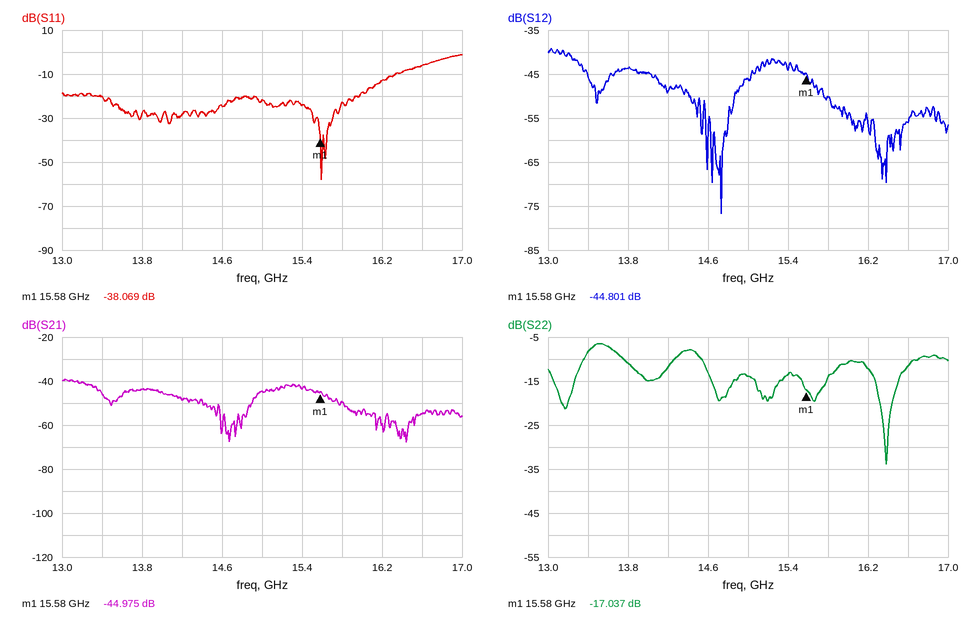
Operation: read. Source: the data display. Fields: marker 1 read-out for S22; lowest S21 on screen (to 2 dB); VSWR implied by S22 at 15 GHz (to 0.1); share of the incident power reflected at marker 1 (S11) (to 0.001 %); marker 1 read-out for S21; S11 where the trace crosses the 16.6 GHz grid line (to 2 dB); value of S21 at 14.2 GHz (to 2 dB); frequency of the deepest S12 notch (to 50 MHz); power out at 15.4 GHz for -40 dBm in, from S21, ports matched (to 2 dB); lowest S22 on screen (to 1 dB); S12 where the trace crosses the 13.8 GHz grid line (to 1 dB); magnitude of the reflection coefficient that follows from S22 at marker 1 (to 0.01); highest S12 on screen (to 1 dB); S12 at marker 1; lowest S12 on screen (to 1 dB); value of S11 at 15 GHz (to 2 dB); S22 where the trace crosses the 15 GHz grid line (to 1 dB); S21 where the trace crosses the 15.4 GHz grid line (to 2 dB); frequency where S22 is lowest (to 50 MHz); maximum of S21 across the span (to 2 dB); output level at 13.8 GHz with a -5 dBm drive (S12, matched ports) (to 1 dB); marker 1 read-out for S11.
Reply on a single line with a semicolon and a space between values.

-17.037 dB; -68 dB; 1.5; 0.016 %; -44.975 dB; -6 dB; -48 dB; 14.75 GHz; -84 dBm; -34 dB; -44 dB; 0.14; -39 dB; -44.801 dB; -77 dB; -22 dB; -14 dB; -44 dB; 16.40 GHz; -40 dB; -49 dBm; -38.069 dB
